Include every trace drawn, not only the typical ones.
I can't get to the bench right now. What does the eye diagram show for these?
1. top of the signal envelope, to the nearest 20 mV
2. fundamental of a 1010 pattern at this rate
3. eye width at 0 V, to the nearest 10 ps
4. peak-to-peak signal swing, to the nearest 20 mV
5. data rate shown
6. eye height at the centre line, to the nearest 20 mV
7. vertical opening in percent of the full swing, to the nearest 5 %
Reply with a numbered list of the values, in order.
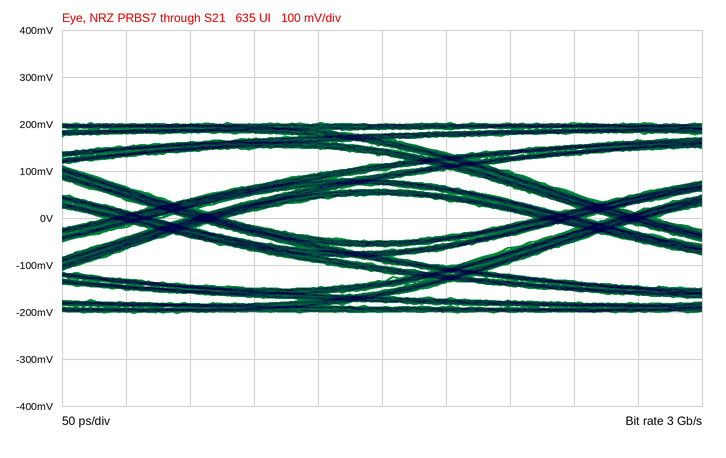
1. 200 mV
2. 1.5 GHz
3. 240 ps
4. 400 mV
5. 3 Gb/s
6. 100 mV
7. 25 %
